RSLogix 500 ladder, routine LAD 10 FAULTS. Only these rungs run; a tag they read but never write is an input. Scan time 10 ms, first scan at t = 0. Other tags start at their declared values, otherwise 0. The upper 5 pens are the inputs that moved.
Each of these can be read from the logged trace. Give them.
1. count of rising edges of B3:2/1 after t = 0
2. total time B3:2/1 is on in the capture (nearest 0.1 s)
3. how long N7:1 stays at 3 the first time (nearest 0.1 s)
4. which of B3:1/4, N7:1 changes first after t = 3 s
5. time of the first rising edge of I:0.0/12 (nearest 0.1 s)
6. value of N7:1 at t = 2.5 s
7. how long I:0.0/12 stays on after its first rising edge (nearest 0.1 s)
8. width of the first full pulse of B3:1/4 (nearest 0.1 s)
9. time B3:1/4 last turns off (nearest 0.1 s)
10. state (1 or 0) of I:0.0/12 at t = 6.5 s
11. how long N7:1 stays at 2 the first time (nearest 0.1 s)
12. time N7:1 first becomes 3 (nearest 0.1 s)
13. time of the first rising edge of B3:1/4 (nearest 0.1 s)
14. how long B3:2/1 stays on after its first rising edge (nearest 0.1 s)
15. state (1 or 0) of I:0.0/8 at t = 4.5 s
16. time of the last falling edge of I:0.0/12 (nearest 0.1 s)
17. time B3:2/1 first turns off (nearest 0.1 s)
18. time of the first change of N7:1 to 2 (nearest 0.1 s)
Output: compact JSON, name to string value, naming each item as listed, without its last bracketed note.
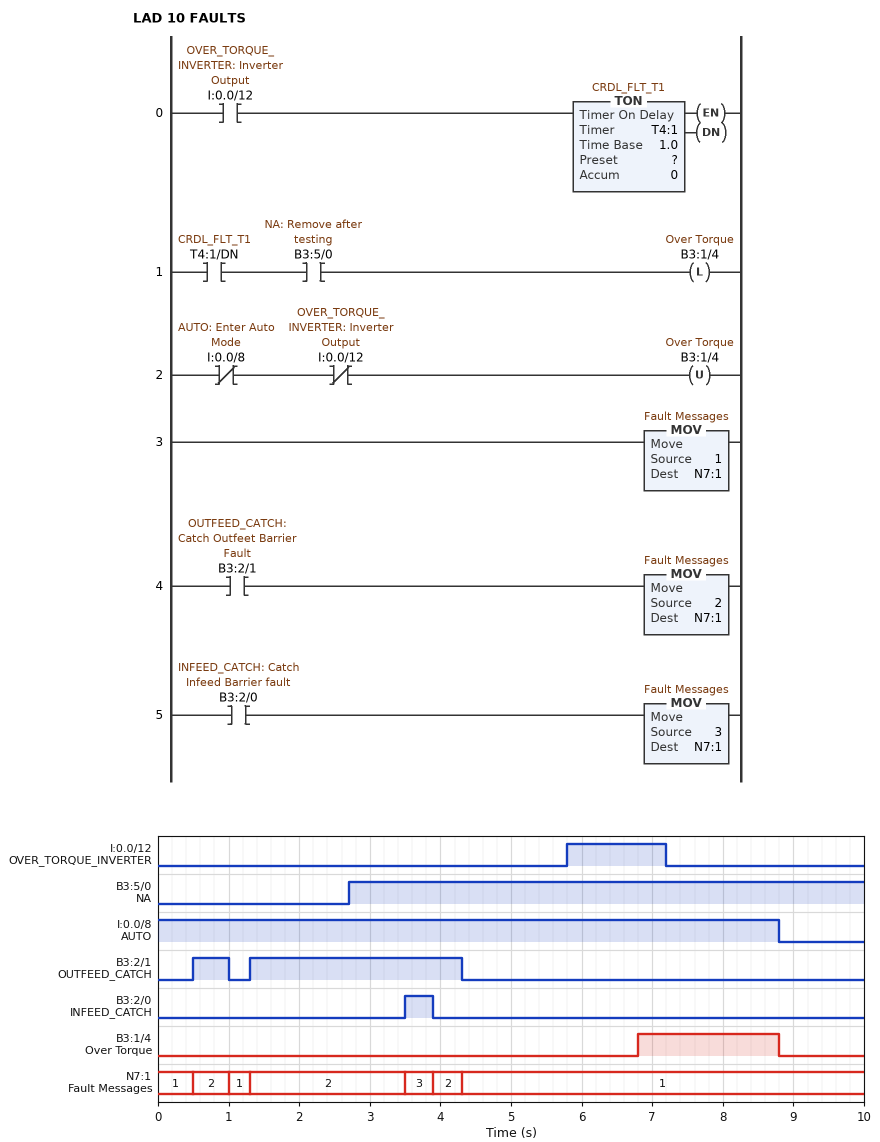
{"count of rising edges of B3:2/1 after t = 0": "2", "total time B3:2/1 is on in the capture": "3.5 s", "how long N7:1 stays at 3 the first time": "0.4 s", "which of B3:1/4, N7:1 changes first after t = 3 s": "N7:1", "time of the first rising edge of I:0.0/12": "5.8 s", "value of N7:1 at t = 2.5 s": "2", "how long I:0.0/12 stays on after its first rising edge": "1.4 s", "width of the first full pulse of B3:1/4": "2.0 s", "time B3:1/4 last turns off": "8.8 s", "state (1 or 0) of I:0.0/12 at t = 6.5 s": "1", "how long N7:1 stays at 2 the first time": "0.5 s", "time N7:1 first becomes 3": "3.5 s", "time of the first rising edge of B3:1/4": "6.8 s", "how long B3:2/1 stays on after its first rising edge": "0.5 s", "state (1 or 0) of I:0.0/8 at t = 4.5 s": "1", "time of the last falling edge of I:0.0/12": "7.2 s", "time B3:2/1 first turns off": "1.0 s", "time of the first change of N7:1 to 2": "0.5 s"}
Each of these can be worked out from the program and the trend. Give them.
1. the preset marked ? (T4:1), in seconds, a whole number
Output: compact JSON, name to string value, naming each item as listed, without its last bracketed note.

{"the preset marked ? (T4:1), in seconds, a whole number": "1 s"}
